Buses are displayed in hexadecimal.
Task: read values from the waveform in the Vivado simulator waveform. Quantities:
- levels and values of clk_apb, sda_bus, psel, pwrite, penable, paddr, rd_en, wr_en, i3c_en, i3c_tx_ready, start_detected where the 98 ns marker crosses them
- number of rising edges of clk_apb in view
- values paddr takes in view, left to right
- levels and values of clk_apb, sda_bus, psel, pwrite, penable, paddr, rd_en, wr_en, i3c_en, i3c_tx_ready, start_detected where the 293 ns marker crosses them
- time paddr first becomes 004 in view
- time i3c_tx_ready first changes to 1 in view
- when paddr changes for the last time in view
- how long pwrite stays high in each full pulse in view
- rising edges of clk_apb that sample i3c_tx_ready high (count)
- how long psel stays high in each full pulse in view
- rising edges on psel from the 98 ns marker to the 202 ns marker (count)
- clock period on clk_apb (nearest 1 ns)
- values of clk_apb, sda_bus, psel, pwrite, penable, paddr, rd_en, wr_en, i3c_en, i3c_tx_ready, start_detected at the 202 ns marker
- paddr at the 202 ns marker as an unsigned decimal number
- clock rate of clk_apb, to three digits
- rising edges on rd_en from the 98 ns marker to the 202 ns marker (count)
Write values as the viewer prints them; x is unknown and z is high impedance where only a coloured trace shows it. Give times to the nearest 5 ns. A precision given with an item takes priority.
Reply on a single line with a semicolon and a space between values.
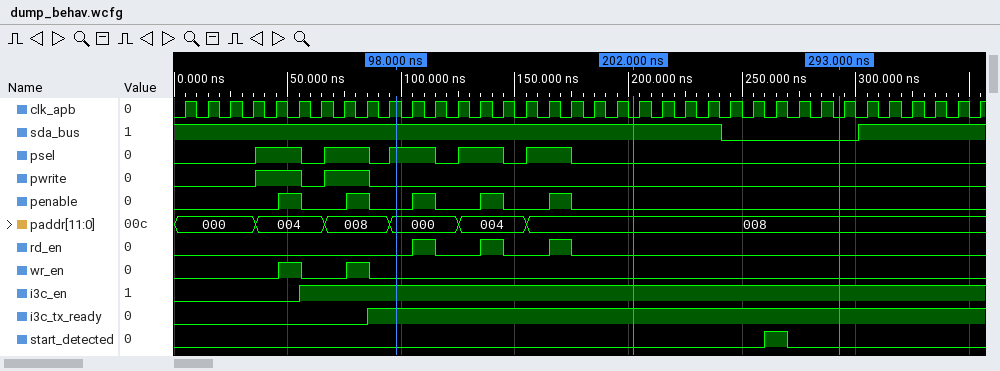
clk_apb=1, sda_bus=1, psel=1, pwrite=0, penable=0, paddr=000, rd_en=0, wr_en=0, i3c_en=1, i3c_tx_ready=1, start_detected=0; 36; 000, 004, 008, 000, 004, 008; clk_apb=0, sda_bus=0, psel=0, pwrite=0, penable=0, paddr=008, rd_en=0, wr_en=0, i3c_en=1, i3c_tx_ready=1, start_detected=0; 35 ns; 85 ns; 155 ns; 20 ns, 20 ns; 27; 20 ns, 20 ns, 20 ns, 20 ns, 20 ns; 2; 10 ns; clk_apb=0, sda_bus=1, psel=0, pwrite=0, penable=0, paddr=008, rd_en=0, wr_en=0, i3c_en=1, i3c_tx_ready=1, start_detected=0; 8; 100 MHz; 3
